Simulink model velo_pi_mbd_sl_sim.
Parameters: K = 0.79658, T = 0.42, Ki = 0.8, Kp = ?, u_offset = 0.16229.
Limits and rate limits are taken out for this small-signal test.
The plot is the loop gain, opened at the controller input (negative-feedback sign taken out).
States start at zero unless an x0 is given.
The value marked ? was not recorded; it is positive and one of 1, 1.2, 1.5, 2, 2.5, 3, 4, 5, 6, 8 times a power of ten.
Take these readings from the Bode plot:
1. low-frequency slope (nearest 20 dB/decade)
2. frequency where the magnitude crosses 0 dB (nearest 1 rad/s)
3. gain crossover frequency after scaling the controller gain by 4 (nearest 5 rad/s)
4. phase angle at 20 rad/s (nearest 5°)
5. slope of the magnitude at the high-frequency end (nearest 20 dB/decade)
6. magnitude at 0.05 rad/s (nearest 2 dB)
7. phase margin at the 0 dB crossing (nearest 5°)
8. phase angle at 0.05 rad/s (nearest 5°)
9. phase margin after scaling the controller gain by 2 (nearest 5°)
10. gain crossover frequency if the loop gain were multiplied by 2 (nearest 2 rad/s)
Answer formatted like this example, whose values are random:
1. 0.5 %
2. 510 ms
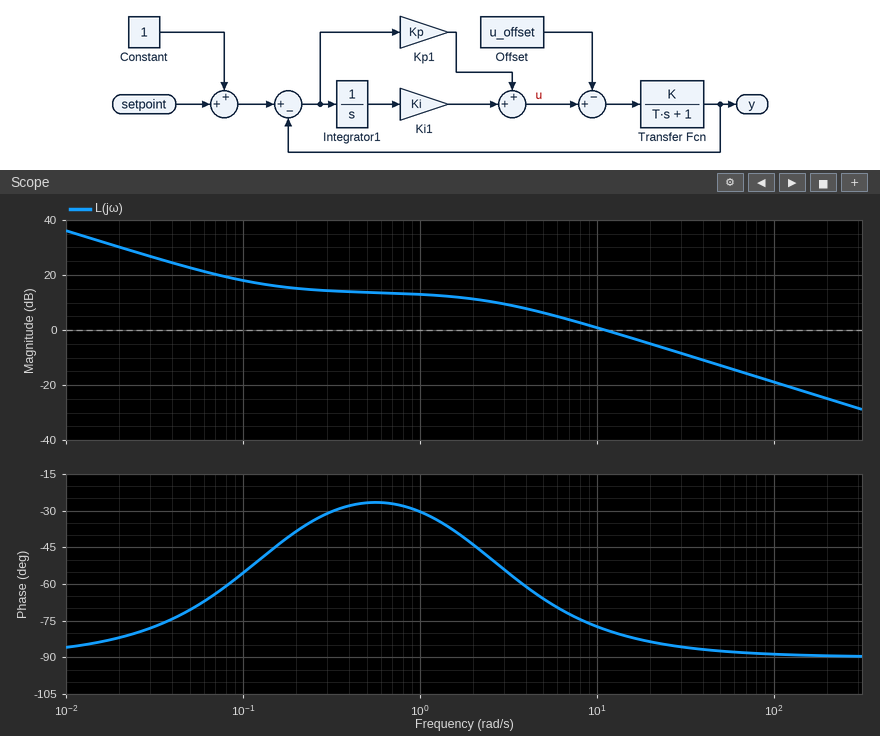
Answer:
1. -20 dB/decade
2. 11 rad/s
3. 45 rad/s
4. -85°
5. -20 dB/decade
6. 22 dB
7. 100°
8. -70°
9. 95°
10. 22 rad/s
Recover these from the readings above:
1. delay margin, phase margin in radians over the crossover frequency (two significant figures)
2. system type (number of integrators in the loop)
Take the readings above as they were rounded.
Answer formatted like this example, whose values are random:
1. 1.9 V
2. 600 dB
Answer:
1. 0.16 s
2. 1
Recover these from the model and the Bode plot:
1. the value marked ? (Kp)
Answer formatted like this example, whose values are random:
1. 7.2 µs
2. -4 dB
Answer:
1. 6
